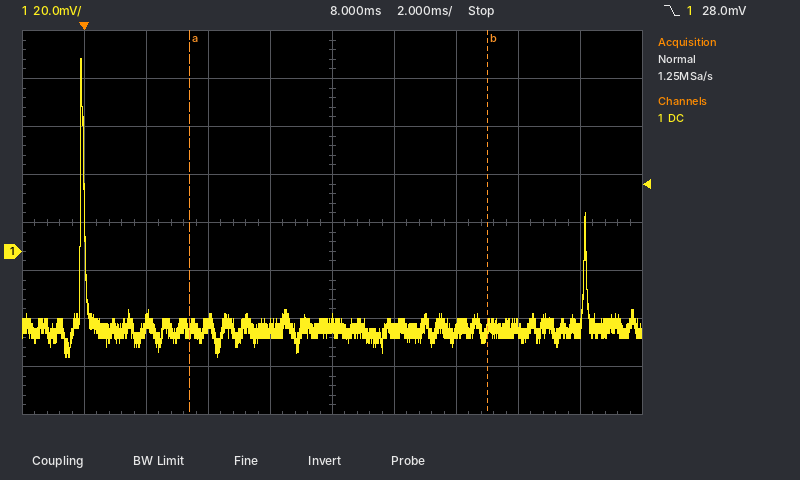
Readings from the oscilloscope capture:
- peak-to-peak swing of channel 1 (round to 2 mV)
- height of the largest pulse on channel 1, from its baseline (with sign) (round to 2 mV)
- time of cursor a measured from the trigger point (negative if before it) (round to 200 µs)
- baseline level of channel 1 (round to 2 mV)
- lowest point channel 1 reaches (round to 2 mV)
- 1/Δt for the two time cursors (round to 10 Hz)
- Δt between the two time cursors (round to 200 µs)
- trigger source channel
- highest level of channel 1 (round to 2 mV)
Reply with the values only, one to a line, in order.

124 mV
+112 mV
+3.4 ms
-32 mV
-44 mV
100 Hz
9.6 ms
channel 1
80 mV
